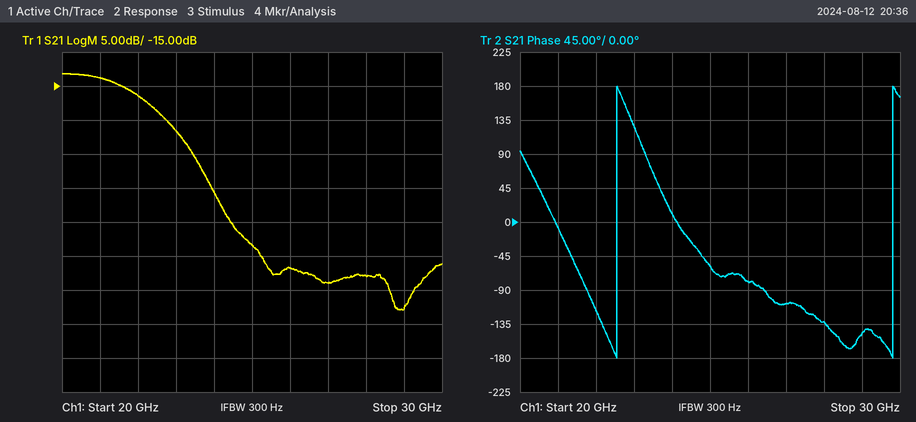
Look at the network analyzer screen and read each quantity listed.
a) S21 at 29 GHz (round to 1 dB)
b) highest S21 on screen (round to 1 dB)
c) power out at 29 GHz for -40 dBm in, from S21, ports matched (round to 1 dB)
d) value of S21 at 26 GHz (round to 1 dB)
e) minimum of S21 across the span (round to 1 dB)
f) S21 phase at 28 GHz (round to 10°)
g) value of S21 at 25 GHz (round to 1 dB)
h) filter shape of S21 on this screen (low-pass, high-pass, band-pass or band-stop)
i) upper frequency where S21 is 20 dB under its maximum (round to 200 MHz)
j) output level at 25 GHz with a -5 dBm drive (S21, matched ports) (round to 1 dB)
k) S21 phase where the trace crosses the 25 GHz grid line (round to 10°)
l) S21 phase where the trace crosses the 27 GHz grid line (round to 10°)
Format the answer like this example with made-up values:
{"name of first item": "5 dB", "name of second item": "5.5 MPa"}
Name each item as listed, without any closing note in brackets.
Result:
{"S21 at 29 GHz": "-48 dB", "highest S21 on screen": "-13 dB", "power out at 29 GHz for -40 dBm in, from S21, ports matched": "-88 dBm", "value of S21 at 26 GHz": "-42 dB", "minimum of S21 across the span": "-48 dB", "S21 phase at 28 GHz": "-130°", "value of S21 at 25 GHz": "-38 dB", "filter shape of S21 on this screen": "low-pass", "upper frequency where S21 is 20 dB under its maximum": "24.2 GHz", "output level at 25 GHz with a -5 dBm drive (S21, matched ports)": "-43 dBm", "S21 phase where the trace crosses the 25 GHz grid line": "-60°", "S21 phase where the trace crosses the 27 GHz grid line": "-110°"}
